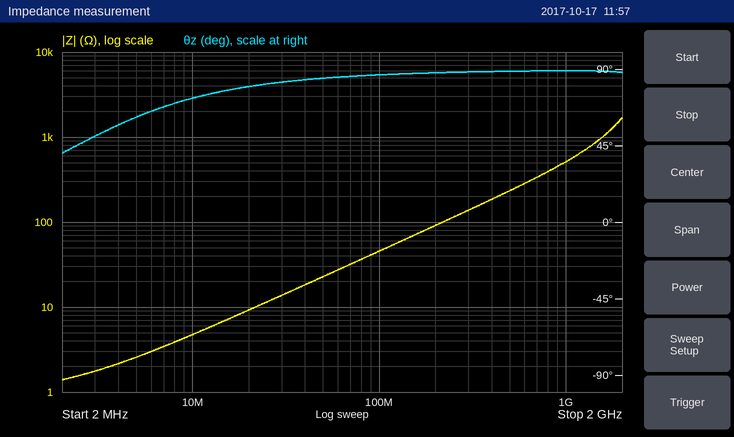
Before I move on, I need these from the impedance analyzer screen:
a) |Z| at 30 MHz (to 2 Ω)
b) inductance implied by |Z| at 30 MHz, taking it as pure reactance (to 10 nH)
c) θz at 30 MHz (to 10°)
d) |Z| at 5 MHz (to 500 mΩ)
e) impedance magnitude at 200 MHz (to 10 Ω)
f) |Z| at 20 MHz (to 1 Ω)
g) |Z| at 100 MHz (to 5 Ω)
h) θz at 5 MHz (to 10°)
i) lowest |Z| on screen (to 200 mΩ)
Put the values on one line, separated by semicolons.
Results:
14 Ω; 70 nH; 80°; 2.5 Ω; 90 Ω; 9 Ω; 45 Ω; 60°; 1.4 Ω
